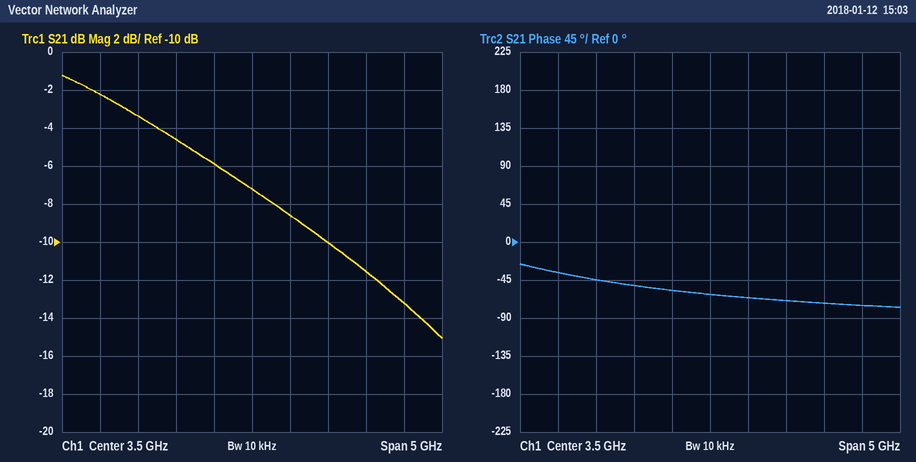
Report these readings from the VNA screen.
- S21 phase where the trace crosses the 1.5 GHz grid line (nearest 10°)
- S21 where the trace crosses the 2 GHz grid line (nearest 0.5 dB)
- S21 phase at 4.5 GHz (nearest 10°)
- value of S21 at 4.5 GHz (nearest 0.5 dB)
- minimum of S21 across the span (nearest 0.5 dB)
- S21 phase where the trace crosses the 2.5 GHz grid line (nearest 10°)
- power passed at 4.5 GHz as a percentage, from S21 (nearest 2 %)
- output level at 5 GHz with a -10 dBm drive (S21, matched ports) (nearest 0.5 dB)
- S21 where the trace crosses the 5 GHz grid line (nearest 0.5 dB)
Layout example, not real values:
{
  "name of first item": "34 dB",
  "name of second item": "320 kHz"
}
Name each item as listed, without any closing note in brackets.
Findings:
{
  "S21 phase where the trace crosses the 1.5 GHz grid line": "-40°",
  "S21 where the trace crosses the 2 GHz grid line": "-3.5 dB",
  "S21 phase at 4.5 GHz": "-70°",
  "value of S21 at 4.5 GHz": "-10.0 dB",
  "minimum of S21 across the span": "-15.0 dB",
  "S21 phase where the trace crosses the 2.5 GHz grid line": "-50°",
  "power passed at 4.5 GHz as a percentage, from S21": "10 %",
  "output level at 5 GHz with a -10 dBm drive (S21, matched ports)": "-21.5 dBm",
  "S21 where the trace crosses the 5 GHz grid line": "-11.5 dB"
}
